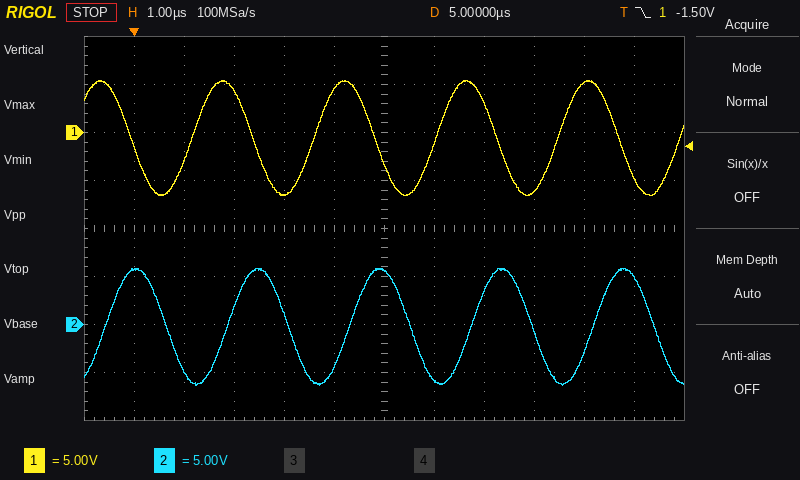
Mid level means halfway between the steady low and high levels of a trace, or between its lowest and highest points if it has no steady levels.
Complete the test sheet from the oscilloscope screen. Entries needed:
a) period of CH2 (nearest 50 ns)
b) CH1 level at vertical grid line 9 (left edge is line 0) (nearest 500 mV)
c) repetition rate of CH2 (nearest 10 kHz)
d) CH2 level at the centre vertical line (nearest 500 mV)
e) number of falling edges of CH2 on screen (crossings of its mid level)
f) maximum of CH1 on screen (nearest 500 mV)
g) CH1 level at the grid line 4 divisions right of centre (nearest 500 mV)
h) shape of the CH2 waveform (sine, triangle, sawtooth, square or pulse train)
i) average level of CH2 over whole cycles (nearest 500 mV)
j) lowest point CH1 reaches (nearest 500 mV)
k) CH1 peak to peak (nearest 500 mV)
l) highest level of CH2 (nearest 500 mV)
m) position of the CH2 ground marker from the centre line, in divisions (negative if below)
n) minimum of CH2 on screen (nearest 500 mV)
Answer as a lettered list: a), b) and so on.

a) 2.45 µs
b) -6.0 V
c) 410 kHz
d) 5.5 V
e) 5
f) 5.5 V
g) 5.0 V
h) sine
i) 0.0 V
j) -6.5 V
k) 12.0 V
l) 6.0 V
m) -2.0 div
n) -6.5 V
